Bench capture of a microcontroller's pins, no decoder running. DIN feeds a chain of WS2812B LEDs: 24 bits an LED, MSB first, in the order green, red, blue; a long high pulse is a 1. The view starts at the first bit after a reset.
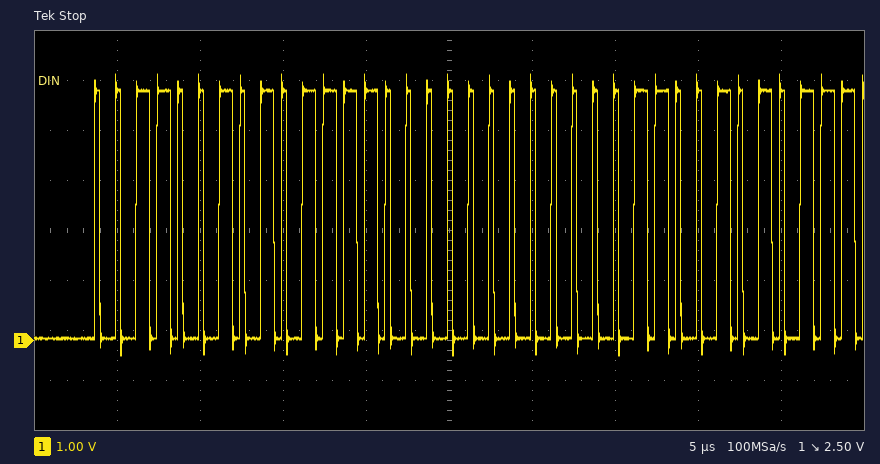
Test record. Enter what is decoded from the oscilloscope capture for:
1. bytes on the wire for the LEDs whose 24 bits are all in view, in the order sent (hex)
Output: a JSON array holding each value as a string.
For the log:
["32 BC 00"]
